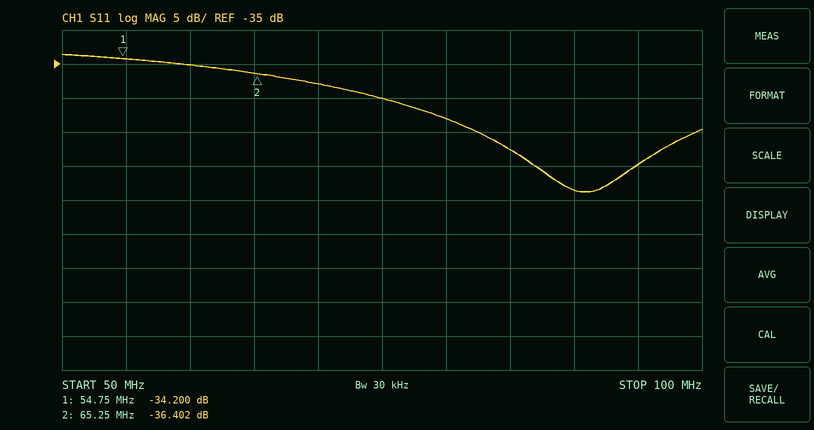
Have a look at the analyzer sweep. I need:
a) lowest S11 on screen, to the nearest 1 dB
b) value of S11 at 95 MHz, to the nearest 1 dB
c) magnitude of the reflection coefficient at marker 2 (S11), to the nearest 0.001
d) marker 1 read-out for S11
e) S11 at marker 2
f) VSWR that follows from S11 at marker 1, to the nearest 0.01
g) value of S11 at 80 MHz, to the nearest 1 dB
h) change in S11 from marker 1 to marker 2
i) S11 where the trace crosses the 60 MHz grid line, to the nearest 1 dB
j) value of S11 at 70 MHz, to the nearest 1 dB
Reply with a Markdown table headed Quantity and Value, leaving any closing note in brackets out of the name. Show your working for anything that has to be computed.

| Quantity | Value |
|---|---|
| lowest S11 on screen, to the nearest 1 dB | -54 dB |
| value of S11 at 95 MHz, to the nearest 1 dB | -50 dB |
| magnitude of the reflection coefficient at marker 2 (S11), to the nearest 0.001 | 10^(-36.402/20) ≈ 0.015 |
| marker 1 read-out for S11 | -34.200 dB |
| S11 at marker 2 | -36.402 dB |
| VSWR that follows from S11 at marker 1, to the nearest 0.01 | (1 + 0.0195)/(1 − 0.0195) ≈ 1.04 |
| value of S11 at 80 MHz, to the nearest 1 dB | -43 dB |
| change in S11 from marker 1 to marker 2 | -36.402 − (-34.2) = -2.202 dB |
| S11 where the trace crosses the 60 MHz grid line, to the nearest 1 dB | -35 dB |
| value of S11 at 70 MHz, to the nearest 1 dB | -38 dB |
